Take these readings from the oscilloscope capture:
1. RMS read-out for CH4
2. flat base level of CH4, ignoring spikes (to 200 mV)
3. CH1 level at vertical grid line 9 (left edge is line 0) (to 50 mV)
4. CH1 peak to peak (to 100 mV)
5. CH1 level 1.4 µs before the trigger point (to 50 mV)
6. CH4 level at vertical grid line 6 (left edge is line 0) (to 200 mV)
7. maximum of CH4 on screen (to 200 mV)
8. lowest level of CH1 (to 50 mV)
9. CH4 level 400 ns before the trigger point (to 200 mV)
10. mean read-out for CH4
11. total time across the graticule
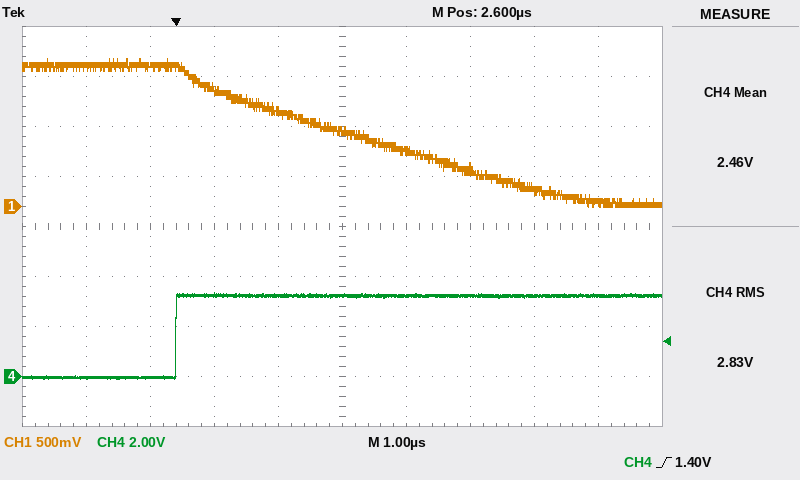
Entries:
2.83 V
0.0 V
50 mV
1.50 V
1.40 V
3.2 V
3.4 V
0 mV
0.0 V
2.46 V
10 µs
